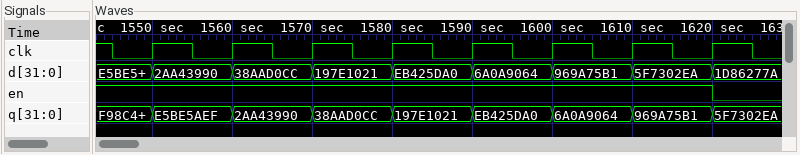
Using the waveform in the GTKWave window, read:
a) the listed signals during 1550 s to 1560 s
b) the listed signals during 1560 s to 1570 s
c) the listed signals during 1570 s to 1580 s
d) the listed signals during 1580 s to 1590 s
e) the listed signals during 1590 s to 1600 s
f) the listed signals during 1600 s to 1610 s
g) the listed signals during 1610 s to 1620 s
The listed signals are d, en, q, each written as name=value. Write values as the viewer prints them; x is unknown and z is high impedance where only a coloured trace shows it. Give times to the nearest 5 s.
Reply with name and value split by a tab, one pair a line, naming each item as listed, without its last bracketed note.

the listed signals during 1550 s to 1560 s	d=2AA43990, en=1, q=E5BE5AEF
the listed signals during 1560 s to 1570 s	d=38AAD0CC, en=1, q=2AA43990
the listed signals during 1570 s to 1580 s	d=197E1021, en=1, q=38AAD0CC
the listed signals during 1580 s to 1590 s	d=EB425DA0, en=1, q=197E1021
the listed signals during 1590 s to 1600 s	d=6A0A9064, en=1, q=EB425DA0
the listed signals during 1600 s to 1610 s	d=969A75B1, en=1, q=6A0A9064
the listed signals during 1610 s to 1620 s	d=5F7302EA, en=1, q=969A75B1
